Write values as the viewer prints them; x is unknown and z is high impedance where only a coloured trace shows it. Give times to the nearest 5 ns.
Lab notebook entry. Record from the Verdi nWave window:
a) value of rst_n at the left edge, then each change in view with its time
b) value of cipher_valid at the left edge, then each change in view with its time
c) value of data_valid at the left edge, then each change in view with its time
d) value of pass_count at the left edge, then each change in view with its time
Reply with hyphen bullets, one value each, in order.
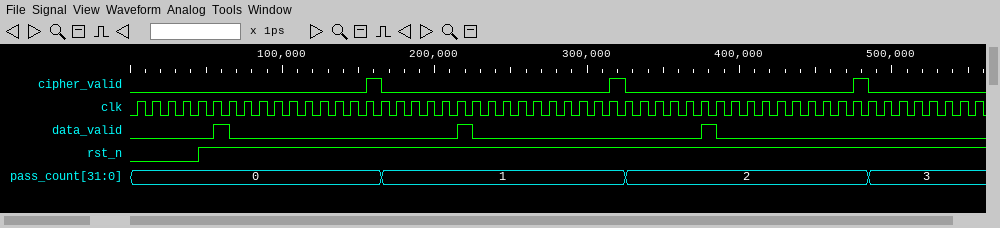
- 0, 1 at 45 ns
- 0, 1 at 155 ns, 0 at 165 ns, 1 at 315 ns, 0 at 325 ns, 1 at 475 ns, 0 at 485 ns
- 0, 1 at 55 ns, 0 at 65 ns, 1 at 215 ns, 0 at 225 ns, 1 at 375 ns, 0 at 385 ns
- 0, 1 at 165 ns, 2 at 325 ns, 3 at 485 ns
